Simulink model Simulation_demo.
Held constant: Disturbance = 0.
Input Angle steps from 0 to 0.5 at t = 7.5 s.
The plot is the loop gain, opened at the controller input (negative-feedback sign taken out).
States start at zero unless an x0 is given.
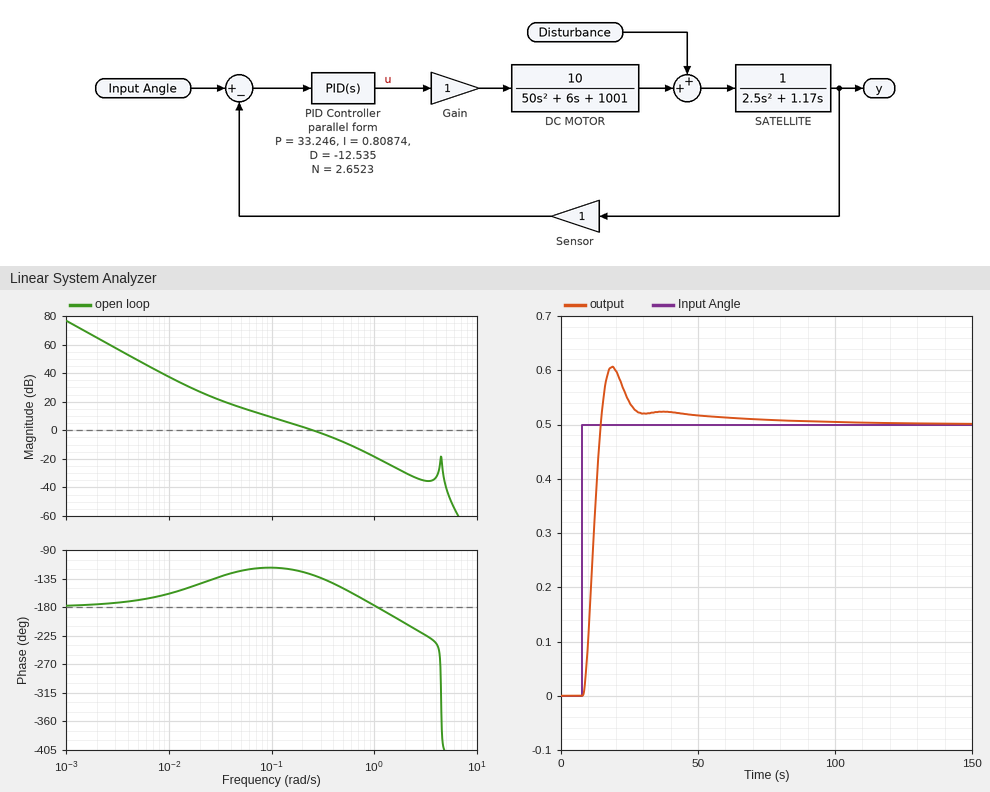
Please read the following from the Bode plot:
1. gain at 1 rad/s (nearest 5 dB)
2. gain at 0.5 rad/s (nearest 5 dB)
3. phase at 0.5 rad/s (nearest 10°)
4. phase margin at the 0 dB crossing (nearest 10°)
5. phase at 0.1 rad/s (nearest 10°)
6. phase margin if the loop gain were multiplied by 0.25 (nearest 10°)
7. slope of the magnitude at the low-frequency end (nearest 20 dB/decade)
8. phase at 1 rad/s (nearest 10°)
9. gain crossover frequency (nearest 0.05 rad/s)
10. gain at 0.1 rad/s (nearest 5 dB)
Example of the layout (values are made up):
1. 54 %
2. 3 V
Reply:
1. -20 dB
2. -10 dB
3. -150°
4. 50°
5. -120°
6. 60°
7. -40 dB/decade
8. -180°
9. 0.25 rad/s
10. 10 dB
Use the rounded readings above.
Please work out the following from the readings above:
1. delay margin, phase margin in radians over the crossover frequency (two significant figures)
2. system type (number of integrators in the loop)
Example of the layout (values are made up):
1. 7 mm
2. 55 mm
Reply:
1. 3.5 s
2. 2
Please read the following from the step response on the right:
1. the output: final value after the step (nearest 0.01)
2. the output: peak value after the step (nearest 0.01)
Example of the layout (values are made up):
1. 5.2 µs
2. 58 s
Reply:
1. 0.50
2. 0.61
